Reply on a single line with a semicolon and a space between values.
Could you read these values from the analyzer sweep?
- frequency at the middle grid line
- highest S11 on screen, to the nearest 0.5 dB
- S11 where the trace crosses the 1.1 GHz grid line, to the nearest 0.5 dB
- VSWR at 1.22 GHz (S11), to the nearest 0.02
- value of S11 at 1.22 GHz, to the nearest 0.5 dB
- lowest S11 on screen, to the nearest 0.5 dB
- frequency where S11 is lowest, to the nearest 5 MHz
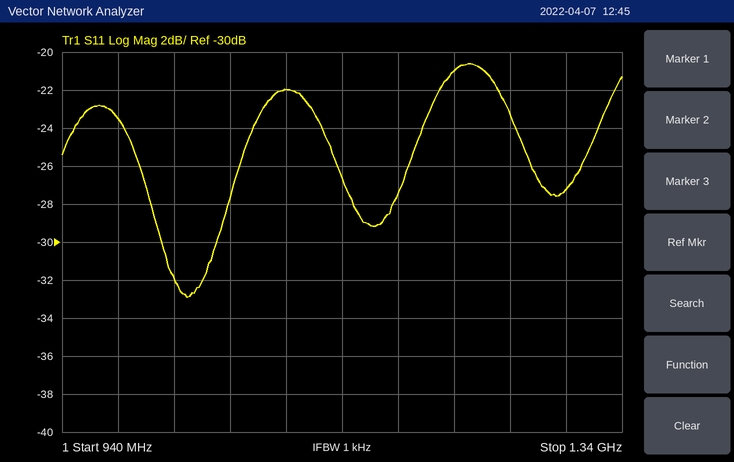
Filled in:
1.14 GHz; -20.5 dB; -22.0 dB; 1.20; -21.0 dB; -33.0 dB; 1.030 GHz
